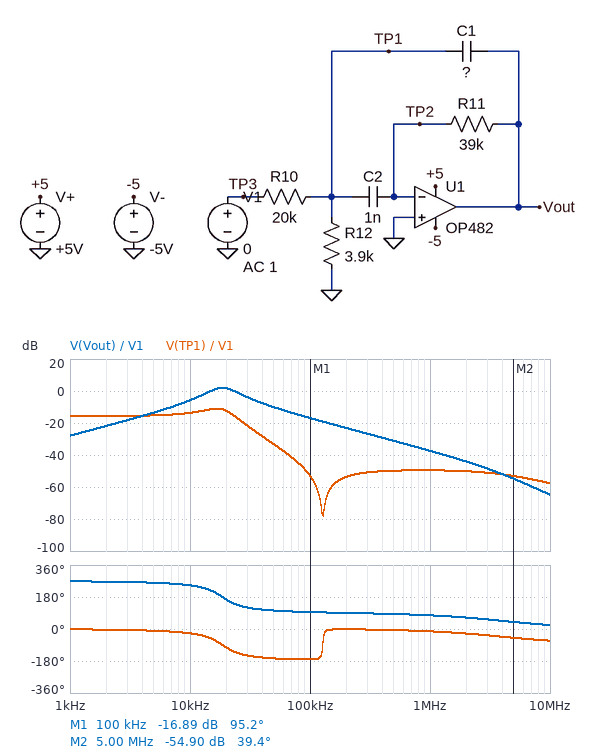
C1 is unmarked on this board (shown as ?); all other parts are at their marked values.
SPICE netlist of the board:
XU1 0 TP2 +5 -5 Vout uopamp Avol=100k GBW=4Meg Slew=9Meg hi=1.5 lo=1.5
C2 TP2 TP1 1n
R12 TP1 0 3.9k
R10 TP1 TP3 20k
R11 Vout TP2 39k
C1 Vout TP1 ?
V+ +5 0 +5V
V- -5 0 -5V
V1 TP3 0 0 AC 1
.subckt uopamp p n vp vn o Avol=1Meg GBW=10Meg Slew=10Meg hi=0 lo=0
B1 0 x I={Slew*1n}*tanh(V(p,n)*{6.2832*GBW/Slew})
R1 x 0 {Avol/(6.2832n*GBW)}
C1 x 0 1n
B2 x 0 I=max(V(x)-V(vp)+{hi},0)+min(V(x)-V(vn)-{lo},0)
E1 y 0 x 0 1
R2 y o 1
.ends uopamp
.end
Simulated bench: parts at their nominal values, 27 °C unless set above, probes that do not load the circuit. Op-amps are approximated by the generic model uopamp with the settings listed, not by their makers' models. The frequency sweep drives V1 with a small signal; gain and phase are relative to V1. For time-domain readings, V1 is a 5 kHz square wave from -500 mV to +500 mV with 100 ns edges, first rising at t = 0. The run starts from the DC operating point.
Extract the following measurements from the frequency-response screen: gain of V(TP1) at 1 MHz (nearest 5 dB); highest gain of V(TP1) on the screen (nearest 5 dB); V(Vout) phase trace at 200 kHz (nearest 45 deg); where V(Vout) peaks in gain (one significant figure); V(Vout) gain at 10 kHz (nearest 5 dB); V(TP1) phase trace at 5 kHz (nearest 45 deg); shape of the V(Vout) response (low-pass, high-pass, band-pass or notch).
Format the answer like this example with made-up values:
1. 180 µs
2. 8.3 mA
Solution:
1. -50 dB
2. -10 dB
3. 90 deg
4. 20 kHz
5. -5 dB
6. 0 deg
7. band-pass
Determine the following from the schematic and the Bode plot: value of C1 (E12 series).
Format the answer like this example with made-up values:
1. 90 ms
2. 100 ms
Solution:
1. 560 pF
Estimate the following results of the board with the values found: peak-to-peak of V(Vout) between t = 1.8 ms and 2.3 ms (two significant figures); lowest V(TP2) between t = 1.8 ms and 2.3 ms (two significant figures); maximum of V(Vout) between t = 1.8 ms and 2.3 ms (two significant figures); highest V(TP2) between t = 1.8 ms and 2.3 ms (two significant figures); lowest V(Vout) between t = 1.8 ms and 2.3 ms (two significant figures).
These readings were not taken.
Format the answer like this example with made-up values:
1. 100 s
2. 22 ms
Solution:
1. 1.0 V
2. -3.4 mV
3. 500 mV
4. 3.4 mV
5. -500 mV
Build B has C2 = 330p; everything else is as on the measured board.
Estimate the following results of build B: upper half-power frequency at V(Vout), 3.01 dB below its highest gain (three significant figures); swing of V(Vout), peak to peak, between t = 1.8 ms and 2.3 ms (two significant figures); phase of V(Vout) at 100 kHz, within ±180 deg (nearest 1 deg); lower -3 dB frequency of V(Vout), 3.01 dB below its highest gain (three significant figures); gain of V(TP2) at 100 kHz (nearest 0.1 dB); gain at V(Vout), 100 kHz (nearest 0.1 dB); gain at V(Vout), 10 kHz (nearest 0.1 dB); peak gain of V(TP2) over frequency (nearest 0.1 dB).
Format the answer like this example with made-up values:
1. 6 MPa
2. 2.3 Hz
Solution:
1. 43.5 kHz
2. 580 mV
3. 101 deg
4. 24.2 kHz
5. -48.4 dB
6. -16.4 dB
7. -16.9 dB
8. -44.2 dB
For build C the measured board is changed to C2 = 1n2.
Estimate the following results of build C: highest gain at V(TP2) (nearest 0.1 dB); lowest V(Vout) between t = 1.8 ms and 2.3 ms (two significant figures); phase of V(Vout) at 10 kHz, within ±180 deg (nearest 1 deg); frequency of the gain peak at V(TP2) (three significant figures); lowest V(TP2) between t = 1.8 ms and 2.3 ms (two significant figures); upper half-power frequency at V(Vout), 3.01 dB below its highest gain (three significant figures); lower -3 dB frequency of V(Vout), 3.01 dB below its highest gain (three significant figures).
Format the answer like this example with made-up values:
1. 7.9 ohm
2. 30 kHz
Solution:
1. -44.5 dB
2. -560 mV
3. -119 deg
4. 18.9 kHz
5. -3.5 mV
6. 23.0 kHz
7. 12.6 kHz
